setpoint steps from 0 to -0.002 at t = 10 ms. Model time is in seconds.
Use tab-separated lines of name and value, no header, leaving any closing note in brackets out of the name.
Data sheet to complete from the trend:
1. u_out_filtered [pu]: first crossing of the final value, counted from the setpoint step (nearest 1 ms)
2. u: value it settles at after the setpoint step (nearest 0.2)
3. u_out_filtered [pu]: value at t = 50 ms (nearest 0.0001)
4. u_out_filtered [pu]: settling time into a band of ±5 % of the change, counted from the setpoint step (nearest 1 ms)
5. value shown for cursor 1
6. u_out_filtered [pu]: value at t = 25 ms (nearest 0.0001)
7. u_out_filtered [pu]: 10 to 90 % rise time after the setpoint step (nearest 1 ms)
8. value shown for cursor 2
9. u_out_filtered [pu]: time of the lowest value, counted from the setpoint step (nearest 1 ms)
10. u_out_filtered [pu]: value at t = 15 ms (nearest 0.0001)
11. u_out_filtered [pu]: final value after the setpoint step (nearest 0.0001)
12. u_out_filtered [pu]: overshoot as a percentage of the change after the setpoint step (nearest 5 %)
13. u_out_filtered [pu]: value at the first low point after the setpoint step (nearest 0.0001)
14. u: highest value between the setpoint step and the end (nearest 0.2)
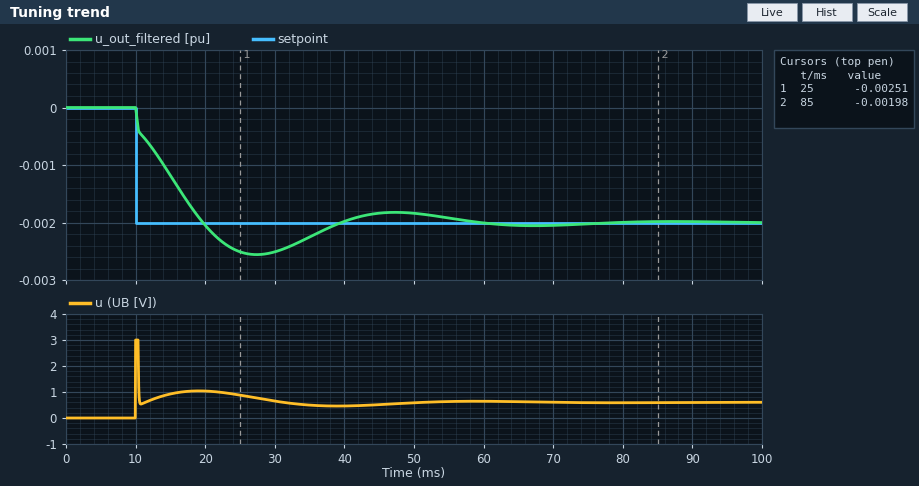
u_out_filtered [pu]: first crossing of the final value, counted from the setpoint step	10 ms
u: value it settles at after the setpoint step	0.6
u_out_filtered [pu]: value at t = 50 ms	-0.0018
u_out_filtered [pu]: settling time into a band of ±5 % of the change, counted from the setpoint step	44 ms
value shown for cursor 1	-0.00251
u_out_filtered [pu]: value at t = 25 ms	-0.0025
u_out_filtered [pu]: 10 to 90 % rise time after the setpoint step	8 ms
value shown for cursor 2	-0.00198
u_out_filtered [pu]: time of the lowest value, counted from the setpoint step	17 ms
u_out_filtered [pu]: value at t = 15 ms	-0.0012
u_out_filtered [pu]: final value after the setpoint step	-0.0020
u_out_filtered [pu]: overshoot as a percentage of the change after the setpoint step	30 %
u_out_filtered [pu]: value at the first low point after the setpoint step	-0.0026
u: highest value between the setpoint step and the end	3.0
